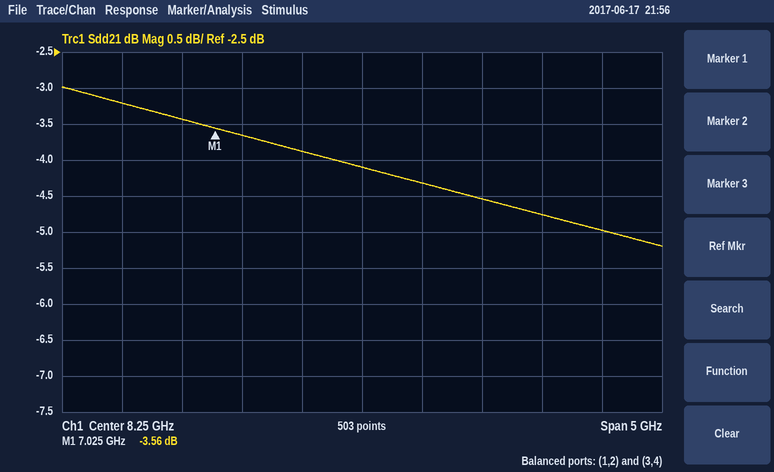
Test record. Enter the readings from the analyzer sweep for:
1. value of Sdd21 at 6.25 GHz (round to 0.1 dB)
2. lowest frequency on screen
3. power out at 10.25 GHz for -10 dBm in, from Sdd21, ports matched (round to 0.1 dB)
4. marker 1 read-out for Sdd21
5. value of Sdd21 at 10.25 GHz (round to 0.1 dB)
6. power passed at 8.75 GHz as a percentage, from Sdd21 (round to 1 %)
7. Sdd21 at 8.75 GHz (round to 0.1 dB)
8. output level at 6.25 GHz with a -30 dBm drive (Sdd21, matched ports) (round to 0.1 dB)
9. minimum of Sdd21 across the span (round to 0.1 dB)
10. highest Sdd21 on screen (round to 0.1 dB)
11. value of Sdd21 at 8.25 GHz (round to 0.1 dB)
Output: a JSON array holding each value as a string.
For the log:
["-3.2 dB", "5.75 GHz", "-15.0 dBm", "-3.56 dB", "-5.0 dB", "37 %", "-4.3 dB", "-33.2 dBm", "-5.2 dB", "-3.0 dB", "-4.1 dB"]
